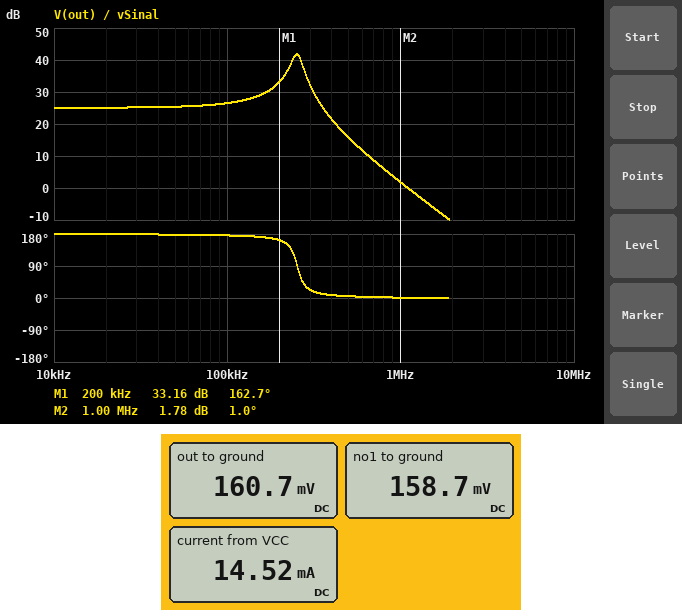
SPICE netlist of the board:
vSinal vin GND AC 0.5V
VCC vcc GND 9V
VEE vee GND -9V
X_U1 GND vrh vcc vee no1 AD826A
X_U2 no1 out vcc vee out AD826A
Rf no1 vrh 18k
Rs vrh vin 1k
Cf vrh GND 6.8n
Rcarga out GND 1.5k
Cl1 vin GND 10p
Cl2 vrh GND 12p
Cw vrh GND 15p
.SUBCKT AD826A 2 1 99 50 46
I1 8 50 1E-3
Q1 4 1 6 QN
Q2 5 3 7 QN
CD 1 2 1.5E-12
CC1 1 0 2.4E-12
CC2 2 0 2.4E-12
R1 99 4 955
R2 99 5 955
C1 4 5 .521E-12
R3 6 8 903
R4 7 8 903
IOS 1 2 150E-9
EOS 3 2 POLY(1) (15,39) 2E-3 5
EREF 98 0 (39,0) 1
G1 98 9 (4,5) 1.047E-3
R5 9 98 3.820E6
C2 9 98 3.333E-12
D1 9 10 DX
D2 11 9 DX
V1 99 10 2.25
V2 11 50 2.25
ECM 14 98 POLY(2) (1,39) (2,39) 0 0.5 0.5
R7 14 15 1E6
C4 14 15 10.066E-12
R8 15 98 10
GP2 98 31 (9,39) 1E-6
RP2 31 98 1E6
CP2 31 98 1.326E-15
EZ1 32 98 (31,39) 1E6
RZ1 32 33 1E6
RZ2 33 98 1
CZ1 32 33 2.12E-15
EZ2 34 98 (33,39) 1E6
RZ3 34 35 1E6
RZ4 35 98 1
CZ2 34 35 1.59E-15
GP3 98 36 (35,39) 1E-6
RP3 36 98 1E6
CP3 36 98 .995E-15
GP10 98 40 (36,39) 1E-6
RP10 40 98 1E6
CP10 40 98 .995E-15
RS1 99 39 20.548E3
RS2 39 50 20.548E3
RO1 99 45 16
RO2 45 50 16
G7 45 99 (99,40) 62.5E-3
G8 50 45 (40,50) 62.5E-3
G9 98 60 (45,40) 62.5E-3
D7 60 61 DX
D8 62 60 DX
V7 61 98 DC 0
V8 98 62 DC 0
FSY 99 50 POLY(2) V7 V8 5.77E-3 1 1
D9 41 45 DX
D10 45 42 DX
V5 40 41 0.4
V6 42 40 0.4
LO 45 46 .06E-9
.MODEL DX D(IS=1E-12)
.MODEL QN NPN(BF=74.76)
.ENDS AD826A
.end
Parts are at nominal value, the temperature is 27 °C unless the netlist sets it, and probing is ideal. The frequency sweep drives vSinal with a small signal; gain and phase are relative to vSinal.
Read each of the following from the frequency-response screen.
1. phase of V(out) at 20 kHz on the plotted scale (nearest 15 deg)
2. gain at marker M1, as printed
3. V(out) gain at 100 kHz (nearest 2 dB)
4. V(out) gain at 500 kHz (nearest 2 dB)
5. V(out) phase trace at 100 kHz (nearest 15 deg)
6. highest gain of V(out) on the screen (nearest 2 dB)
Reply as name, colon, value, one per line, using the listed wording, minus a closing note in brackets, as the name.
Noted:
phase of V(out) at 20 kHz on the plotted scale: 180 deg
gain at marker M1, as printed: 33.16 dB
V(out) gain at 100 kHz: 26 dB
V(out) gain at 500 kHz: 16 dB
V(out) phase trace at 100 kHz: 180 deg
highest gain of V(out) on the screen: 42 dB
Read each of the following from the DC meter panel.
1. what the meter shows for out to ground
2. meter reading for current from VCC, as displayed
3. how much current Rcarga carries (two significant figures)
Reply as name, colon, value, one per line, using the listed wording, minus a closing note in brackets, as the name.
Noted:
what the meter shows for out to ground: 160.7 mV
meter reading for current from VCC, as displayed: 14.52 mA
how much current Rcarga carries: 110 µA
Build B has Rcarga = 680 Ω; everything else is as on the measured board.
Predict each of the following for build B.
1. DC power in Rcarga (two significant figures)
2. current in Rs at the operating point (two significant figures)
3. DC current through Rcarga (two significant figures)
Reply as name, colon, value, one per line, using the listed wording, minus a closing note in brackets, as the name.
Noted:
DC power in Rcarga: 38 µW
current in Rs at the operating point: 2.0 µA
DC current through Rcarga: 240 µA
